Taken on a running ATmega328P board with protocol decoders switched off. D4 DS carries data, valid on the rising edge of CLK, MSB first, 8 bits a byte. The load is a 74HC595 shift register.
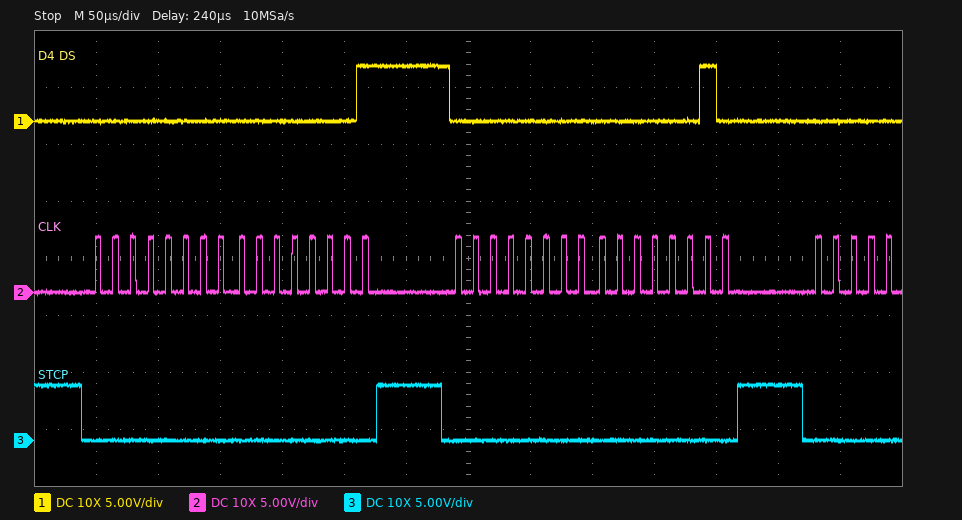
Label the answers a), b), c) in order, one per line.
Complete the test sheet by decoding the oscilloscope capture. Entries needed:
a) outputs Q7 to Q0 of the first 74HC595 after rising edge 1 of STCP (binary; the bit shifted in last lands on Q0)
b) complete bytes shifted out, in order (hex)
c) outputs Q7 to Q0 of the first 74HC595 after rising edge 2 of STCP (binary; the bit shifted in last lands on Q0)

a) 00000001
b) 00 01 00 02
c) 00000010
